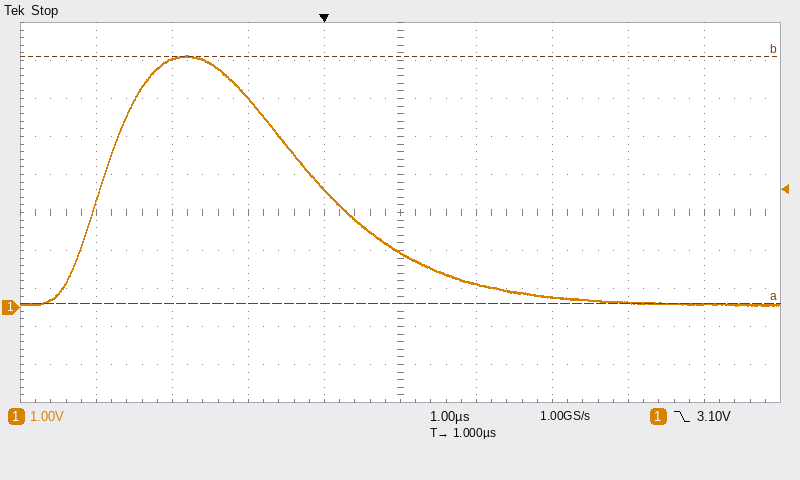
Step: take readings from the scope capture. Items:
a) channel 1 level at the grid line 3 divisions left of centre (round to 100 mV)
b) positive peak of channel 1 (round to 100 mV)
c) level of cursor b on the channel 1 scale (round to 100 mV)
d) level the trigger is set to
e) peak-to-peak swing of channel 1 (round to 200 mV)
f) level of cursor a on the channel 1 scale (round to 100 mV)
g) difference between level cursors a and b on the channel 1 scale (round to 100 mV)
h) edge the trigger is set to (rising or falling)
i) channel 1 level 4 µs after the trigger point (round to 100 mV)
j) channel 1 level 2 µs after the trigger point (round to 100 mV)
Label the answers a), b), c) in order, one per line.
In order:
a) 6.5 V
b) 6.6 V
c) 6.6 V
d) 3.10 V
e) 6.6 V
f) 100 mV
g) 6.5 V
h) falling
i) 100 mV
j) 600 mV
